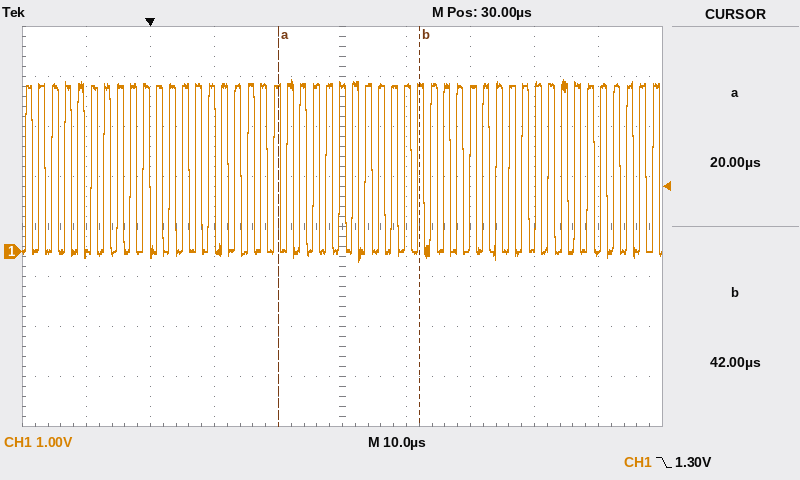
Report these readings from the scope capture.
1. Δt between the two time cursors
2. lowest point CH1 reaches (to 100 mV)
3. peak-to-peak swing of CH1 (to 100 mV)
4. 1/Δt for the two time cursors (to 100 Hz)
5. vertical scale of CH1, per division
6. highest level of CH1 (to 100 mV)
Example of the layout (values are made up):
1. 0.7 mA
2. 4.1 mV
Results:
1. 22 µs
2. -200 mV
3. 3.6 V
4. 45.5 kHz
5. 1 V
6. 3.4 V
